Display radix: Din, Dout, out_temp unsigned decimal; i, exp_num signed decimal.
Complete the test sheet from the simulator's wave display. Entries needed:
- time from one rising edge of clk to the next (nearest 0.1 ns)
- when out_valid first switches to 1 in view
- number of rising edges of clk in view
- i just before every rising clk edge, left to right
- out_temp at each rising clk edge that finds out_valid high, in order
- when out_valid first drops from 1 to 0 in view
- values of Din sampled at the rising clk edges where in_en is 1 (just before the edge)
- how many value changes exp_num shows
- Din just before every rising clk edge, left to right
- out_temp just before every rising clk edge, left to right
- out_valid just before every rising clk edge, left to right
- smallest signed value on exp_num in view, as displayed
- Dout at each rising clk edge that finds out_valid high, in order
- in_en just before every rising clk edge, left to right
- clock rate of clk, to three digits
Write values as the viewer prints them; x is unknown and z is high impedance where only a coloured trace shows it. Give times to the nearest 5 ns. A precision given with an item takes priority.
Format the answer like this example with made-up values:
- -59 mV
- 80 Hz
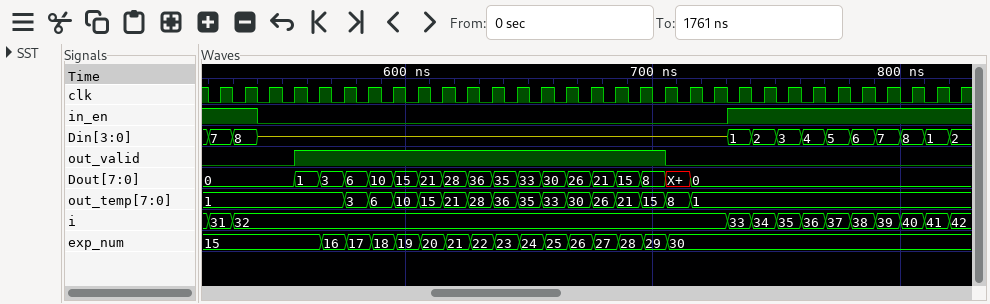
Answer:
- 10 ns
- 555 ns
- 31
- 31, 32, 32, 32, 32, 32, 32, 32, 32, 32, 32, 32, 32, 32, 32, 32, 32, 32, 32, 32, 32, 33, 34, 35, 36, 37, 38, 39, 40, 41, 42
- 1, 1, 3, 6, 10, 15, 21, 28, 36, 35, 33, 30, 26, 21, 15
- 705 ns
- 7, 8, 1, 2, 3, 4, 5, 6, 7, 8, 1, 2
- 15
- 7, 8, z, z, z, z, z, z, z, z, z, z, z, z, z, z, z, z, z, z, z, 1, 2, 3, 4, 5, 6, 7, 8, 1, 2
- 1, 1, 1, 1, 1, 1, 3, 6, 10, 15, 21, 28, 36, 35, 33, 30, 26, 21, 15, 8, 1, 1, 1, 1, 1, 1, 1, 1, 1, 1, 1
- 0 0 0 0 1 1 1 1 1 1 1 1 1 1 1 1 1 1 1 0 0 0 0 0 0 0 0 0 0 0 0
- 15
- 1, 3, 6, 10, 15, 21, 28, 36, 35, 33, 30, 26, 21, 15, 8
- 1 1 0 0 0 0 0 0 0 0 0 0 0 0 0 0 0 0 0 0 0 1 1 1 1 1 1 1 1 1 1
- 100 MHz
